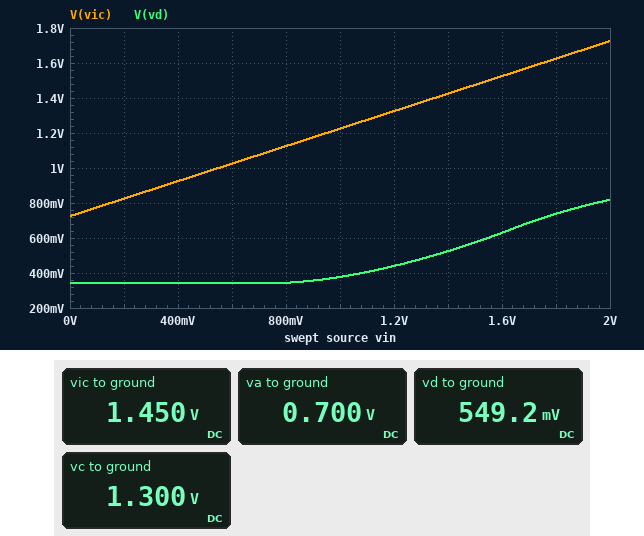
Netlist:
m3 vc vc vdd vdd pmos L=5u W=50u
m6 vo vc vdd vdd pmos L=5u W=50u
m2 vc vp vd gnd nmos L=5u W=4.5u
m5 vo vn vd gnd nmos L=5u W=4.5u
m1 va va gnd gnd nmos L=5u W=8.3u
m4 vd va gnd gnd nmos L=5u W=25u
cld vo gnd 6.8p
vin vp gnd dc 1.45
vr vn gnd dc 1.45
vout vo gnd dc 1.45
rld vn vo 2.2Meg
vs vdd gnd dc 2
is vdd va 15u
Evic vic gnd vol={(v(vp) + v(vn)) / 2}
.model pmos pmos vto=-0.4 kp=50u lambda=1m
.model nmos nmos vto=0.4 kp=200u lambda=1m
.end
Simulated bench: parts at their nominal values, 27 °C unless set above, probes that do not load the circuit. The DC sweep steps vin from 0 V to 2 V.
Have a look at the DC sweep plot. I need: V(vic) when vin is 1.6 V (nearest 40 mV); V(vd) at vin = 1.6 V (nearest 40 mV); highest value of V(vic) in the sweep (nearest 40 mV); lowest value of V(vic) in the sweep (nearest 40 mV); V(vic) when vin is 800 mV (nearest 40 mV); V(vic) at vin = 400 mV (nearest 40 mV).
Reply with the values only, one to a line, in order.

1.52 V
640 mV
1.72 V
720 mV
1.12 V
920 mV
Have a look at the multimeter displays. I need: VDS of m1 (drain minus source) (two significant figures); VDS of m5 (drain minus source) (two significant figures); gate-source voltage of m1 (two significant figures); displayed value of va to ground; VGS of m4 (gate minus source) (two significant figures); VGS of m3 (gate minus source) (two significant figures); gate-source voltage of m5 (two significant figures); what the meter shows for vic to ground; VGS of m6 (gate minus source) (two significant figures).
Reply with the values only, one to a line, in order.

700 mV
900 mV
700 mV
0.700 V
700 mV
-700 mV
900 mV
1.450 V
-700 mV
